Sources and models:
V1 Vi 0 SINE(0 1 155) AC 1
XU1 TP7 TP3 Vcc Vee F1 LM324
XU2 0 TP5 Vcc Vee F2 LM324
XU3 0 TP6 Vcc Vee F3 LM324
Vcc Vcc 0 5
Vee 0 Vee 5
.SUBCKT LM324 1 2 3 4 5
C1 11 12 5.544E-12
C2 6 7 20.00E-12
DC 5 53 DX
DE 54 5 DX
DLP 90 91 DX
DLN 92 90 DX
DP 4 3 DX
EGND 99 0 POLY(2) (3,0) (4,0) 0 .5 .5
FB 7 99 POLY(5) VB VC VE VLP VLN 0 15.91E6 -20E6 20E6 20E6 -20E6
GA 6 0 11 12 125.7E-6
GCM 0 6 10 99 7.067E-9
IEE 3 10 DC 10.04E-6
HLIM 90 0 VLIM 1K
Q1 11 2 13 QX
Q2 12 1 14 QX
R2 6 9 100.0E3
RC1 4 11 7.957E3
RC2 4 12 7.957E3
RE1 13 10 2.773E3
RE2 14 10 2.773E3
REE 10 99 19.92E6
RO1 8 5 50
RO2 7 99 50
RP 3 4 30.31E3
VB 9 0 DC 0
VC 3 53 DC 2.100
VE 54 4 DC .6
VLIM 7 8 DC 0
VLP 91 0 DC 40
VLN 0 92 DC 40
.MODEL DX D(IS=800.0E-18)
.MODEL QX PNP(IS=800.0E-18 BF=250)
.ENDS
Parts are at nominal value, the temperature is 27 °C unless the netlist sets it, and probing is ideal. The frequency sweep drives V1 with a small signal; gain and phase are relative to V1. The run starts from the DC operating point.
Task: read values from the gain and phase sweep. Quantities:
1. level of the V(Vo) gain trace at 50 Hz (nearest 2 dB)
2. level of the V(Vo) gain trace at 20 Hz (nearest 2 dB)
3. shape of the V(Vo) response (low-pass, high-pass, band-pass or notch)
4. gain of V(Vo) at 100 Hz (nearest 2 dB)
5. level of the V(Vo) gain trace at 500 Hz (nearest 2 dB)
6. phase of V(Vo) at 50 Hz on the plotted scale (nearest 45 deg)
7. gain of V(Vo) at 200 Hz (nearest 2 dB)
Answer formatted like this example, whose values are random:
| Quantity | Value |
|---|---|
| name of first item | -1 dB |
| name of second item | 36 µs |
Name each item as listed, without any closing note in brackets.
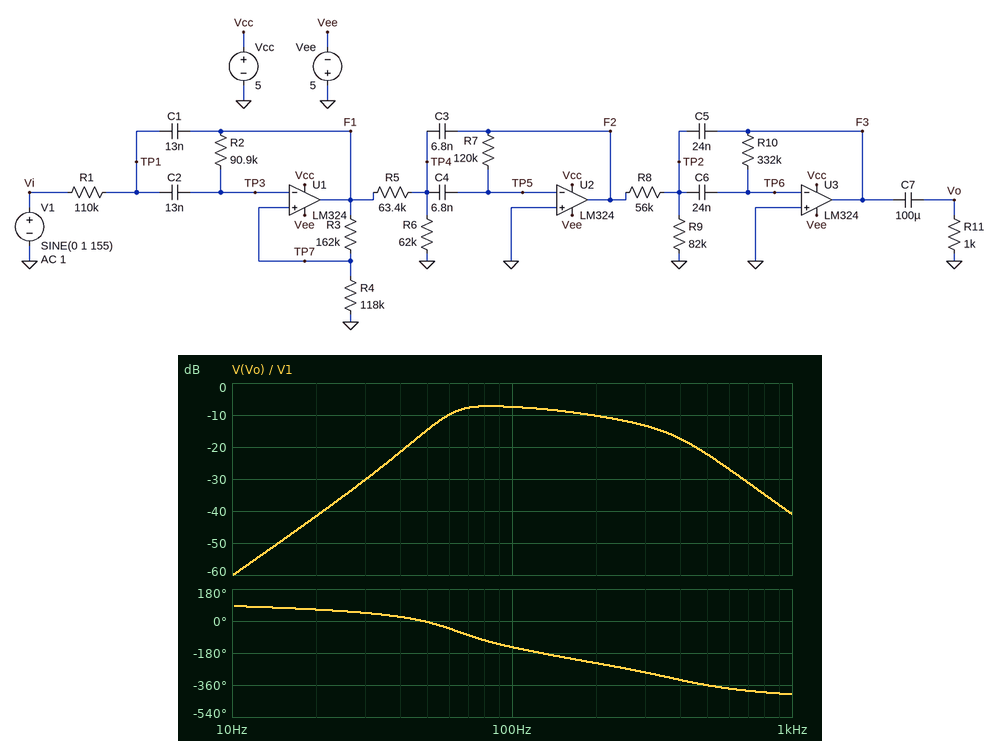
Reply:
| Quantity | Value |
|---|---|
| level of the V(Vo) gain trace at 50 Hz | -14 dB |
| level of the V(Vo) gain trace at 20 Hz | -42 dB |
| shape of the V(Vo) response | band-pass |
| gain of V(Vo) at 100 Hz | -8 dB |
| level of the V(Vo) gain trace at 500 Hz | -22 dB |
| phase of V(Vo) at 50 Hz on the plotted scale | 0 deg |
| gain of V(Vo) at 200 Hz | -10 dB |
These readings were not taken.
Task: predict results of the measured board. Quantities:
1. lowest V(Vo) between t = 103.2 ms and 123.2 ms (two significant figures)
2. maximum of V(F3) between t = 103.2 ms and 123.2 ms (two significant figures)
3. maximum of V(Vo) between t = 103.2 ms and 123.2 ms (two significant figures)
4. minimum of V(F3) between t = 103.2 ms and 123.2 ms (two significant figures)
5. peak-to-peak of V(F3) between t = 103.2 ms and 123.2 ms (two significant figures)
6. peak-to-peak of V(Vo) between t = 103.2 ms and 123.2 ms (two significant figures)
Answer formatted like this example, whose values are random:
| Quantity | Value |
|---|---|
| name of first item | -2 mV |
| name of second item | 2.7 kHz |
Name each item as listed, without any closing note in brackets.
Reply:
| Quantity | Value |
|---|---|
| lowest V(Vo) between t = 103.2 ms and 123.2 ms | -360 mV |
| maximum of V(F3) between t = 103.2 ms and 123.2 ms | 350 mV |
| maximum of V(Vo) between t = 103.2 ms and 123.2 ms | 360 mV |
| minimum of V(F3) between t = 103.2 ms and 123.2 ms | -370 mV |
| peak-to-peak of V(F3) between t = 103.2 ms and 123.2 ms | 720 mV |
| peak-to-peak of V(Vo) between t = 103.2 ms and 123.2 ms | 720 mV |
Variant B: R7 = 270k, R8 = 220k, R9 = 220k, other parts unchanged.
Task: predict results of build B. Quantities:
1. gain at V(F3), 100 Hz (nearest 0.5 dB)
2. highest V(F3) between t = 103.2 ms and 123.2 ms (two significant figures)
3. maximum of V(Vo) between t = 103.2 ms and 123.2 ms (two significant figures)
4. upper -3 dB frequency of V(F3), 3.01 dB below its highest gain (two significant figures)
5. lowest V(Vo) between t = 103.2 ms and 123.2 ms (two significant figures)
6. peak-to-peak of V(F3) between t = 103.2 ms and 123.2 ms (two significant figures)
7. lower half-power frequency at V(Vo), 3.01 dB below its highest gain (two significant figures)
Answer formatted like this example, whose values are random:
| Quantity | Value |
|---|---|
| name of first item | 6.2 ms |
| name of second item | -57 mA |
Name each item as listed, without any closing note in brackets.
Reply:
| Quantity | Value |
|---|---|
| gain at V(F3), 100 Hz | -14.0 dB |
| highest V(F3) between t = 103.2 ms and 123.2 ms | 220 mV |
| maximum of V(Vo) between t = 103.2 ms and 123.2 ms | 230 mV |
| upper -3 dB frequency of V(F3), 3.01 dB below its highest gain | 270 Hz |
| lowest V(Vo) between t = 103.2 ms and 123.2 ms | -230 mV |
| peak-to-peak of V(F3) between t = 103.2 ms and 123.2 ms | 450 mV |
| lower half-power frequency at V(Vo), 3.01 dB below its highest gain | 73 Hz |
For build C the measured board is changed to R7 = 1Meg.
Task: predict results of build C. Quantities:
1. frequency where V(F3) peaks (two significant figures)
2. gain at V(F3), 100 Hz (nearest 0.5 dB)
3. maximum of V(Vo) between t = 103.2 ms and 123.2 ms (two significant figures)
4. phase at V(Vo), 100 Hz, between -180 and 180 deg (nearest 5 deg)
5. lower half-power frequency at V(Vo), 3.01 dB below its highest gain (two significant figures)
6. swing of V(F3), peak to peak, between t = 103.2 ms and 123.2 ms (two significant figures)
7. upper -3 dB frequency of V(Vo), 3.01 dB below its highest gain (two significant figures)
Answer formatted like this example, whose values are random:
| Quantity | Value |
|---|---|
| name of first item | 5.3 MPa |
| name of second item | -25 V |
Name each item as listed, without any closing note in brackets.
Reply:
| Quantity | Value |
|---|---|
| frequency where V(F3) peaks | 130 Hz |
| gain at V(F3), 100 Hz | 16.5 dB |
| maximum of V(Vo) between t = 103.2 ms and 123.2 ms | 3.5 V |
| phase at V(Vo), 100 Hz, between -180 and 180 deg | -165 deg |
| lower half-power frequency at V(Vo), 3.01 dB below its highest gain | 95 Hz |
| swing of V(F3), peak to peak, between t = 103.2 ms and 123.2 ms | 7.1 V |
| upper -3 dB frequency of V(Vo), 3.01 dB below its highest gain | 150 Hz |
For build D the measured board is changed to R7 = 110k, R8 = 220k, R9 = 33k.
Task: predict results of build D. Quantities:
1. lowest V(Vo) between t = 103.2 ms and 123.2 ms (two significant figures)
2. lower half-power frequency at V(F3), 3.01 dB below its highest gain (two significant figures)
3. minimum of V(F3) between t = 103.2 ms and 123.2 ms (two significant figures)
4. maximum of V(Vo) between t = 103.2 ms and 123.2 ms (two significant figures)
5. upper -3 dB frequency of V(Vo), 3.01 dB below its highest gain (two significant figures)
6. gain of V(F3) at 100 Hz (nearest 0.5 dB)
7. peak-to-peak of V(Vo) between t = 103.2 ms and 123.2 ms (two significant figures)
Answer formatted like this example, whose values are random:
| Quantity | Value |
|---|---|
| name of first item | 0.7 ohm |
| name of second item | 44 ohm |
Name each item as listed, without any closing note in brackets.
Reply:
| Quantity | Value |
|---|---|
| lowest V(Vo) between t = 103.2 ms and 123.2 ms | -85 mV |
| lower half-power frequency at V(F3), 3.01 dB below its highest gain | 62 Hz |
| minimum of V(F3) between t = 103.2 ms and 123.2 ms | -92 mV |
| maximum of V(Vo) between t = 103.2 ms and 123.2 ms | 85 mV |
| upper -3 dB frequency of V(Vo), 3.01 dB below its highest gain | 180 Hz |
| gain of V(F3) at 100 Hz | -19.5 dB |
| peak-to-peak of V(Vo) between t = 103.2 ms and 123.2 ms | 170 mV |
